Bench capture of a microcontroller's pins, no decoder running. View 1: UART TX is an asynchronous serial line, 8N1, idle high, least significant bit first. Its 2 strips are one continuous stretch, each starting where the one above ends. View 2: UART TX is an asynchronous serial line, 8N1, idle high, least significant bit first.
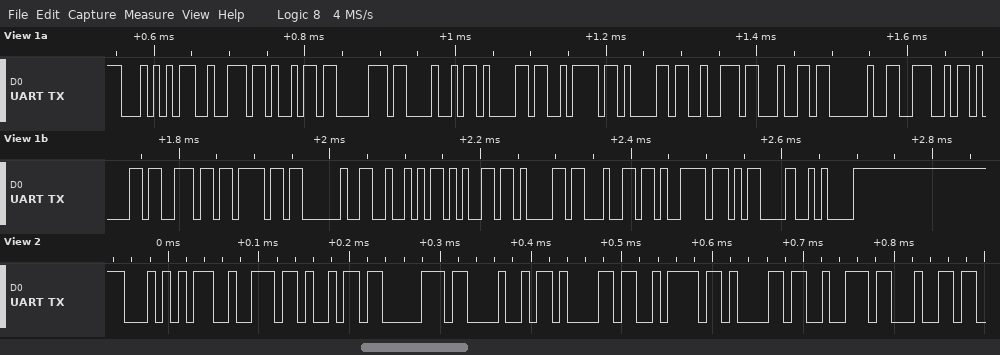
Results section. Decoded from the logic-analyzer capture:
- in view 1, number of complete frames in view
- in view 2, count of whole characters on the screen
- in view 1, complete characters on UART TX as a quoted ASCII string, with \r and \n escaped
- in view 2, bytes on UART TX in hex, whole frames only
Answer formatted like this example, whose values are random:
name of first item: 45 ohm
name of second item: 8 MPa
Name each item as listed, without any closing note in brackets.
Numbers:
in view 1, number of complete frames in view: 23
in view 2, count of whole characters on the screen: 10
in view 1, complete characters on UART TX as a quoted ASCII string, with \r and \n escaped: "TripHazard Nano Ready\r\n"
in view 2, bytes on UART TX in hex, whole frames only: 0x54 0x72 0x69 0x70 0x48 0x61 0x7A 0x61 0x72 0x64
